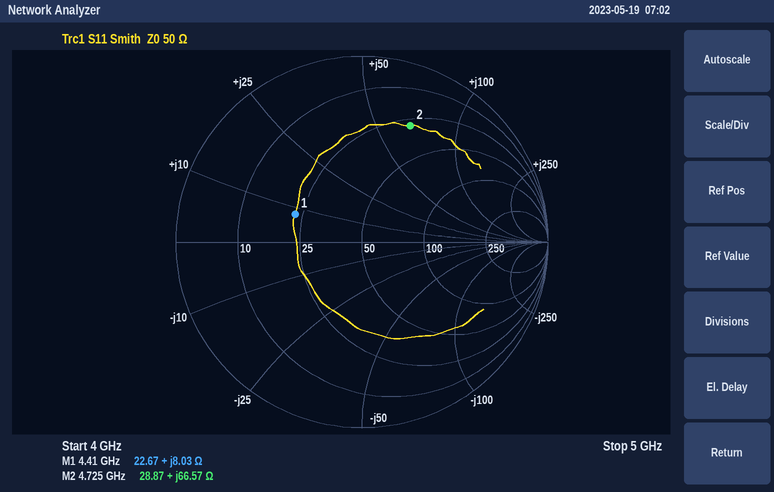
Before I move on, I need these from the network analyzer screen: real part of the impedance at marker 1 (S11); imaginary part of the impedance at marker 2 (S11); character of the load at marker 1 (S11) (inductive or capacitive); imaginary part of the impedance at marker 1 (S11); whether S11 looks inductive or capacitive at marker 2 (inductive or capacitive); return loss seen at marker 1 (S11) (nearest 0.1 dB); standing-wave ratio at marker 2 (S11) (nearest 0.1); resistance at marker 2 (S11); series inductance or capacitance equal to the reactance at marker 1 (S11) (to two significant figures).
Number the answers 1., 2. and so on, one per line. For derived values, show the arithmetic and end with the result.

1. 22.67 Ω
2. +66.57 Ω
3. inductive
4. +8.03 Ω
5. inductive
6. 8.2 dB
7. 5.2
8. 28.87 Ω
9. L = 8.03 Ω/(2π × 4.41 GHz) ≈ 290 pH
